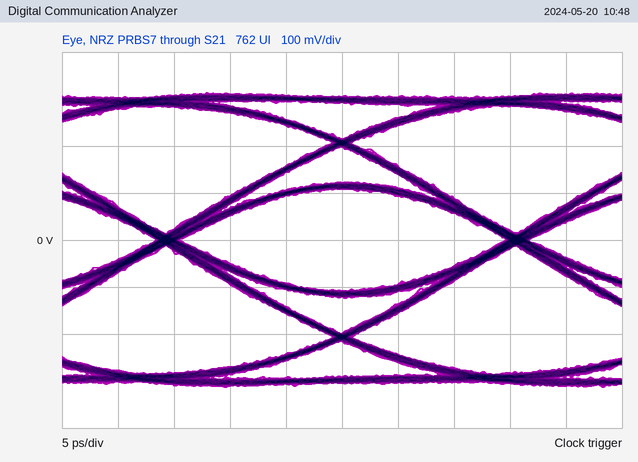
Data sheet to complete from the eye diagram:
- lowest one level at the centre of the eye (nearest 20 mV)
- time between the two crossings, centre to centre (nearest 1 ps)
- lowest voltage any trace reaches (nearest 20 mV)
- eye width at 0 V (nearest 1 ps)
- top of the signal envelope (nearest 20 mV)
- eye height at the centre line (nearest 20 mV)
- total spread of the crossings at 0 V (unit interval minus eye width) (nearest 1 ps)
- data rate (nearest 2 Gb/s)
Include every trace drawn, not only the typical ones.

100 mV
31 ps
-320 mV
29 ps
320 mV
220 mV
2 ps
32 Gb/s
